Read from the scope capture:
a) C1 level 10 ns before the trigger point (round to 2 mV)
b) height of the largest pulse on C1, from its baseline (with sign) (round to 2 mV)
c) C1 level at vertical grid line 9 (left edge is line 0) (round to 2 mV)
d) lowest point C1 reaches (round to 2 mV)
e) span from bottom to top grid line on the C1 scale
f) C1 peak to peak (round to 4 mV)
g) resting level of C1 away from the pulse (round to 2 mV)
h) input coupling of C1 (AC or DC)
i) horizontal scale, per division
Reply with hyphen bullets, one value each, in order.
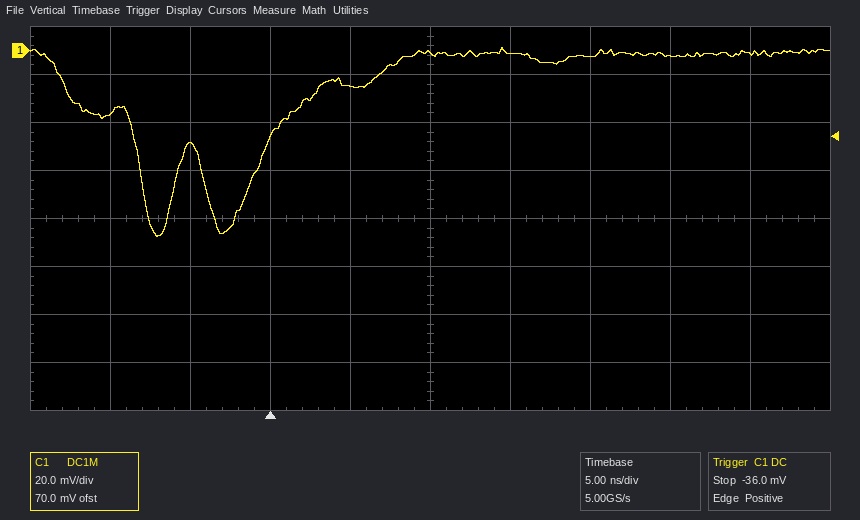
- -26 mV
- -76 mV
- -2 mV
- -78 mV
- 160 mV
- 80 mV
- -2 mV
- DC
- 5 ns
